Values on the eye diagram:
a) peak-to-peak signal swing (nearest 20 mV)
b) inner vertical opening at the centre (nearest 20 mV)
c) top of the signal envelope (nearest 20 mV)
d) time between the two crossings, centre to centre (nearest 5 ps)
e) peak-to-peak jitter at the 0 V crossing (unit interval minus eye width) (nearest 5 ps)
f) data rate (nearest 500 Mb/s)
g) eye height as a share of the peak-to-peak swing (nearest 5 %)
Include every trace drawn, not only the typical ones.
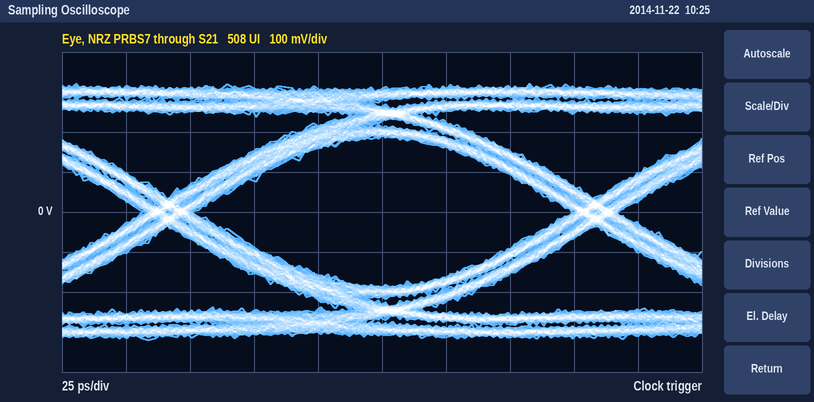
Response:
640 mV
380 mV
320 mV
165 ps
20 ps
6.0 Gb/s
60 %
